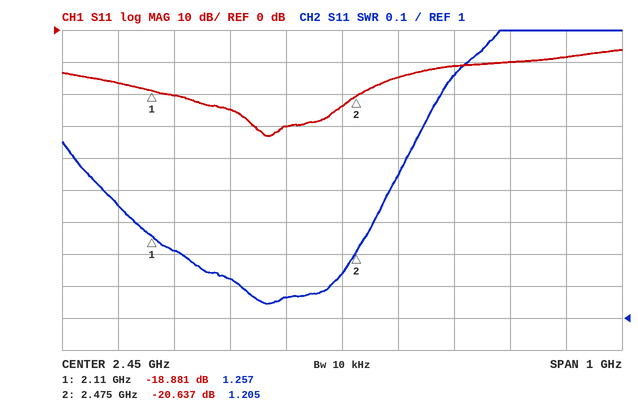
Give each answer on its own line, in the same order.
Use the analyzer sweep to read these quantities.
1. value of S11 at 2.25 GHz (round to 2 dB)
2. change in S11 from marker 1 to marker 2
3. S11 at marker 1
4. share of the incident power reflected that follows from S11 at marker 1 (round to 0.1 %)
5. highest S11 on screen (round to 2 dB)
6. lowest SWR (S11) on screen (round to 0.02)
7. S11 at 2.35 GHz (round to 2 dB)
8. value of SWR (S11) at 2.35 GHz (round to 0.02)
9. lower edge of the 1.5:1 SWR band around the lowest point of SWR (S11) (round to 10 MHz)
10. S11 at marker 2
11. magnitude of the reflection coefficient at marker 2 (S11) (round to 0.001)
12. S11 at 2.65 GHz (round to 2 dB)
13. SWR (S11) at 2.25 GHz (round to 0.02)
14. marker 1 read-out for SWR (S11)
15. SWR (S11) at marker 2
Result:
-24 dB
-1.756 dB
-18.881 dB
1.3 %
-6 dB
1.04
-30 dB
1.06
1.97 GHz
-20.637 dB
0.093
-12 dB
1.12
1.257
1.205
